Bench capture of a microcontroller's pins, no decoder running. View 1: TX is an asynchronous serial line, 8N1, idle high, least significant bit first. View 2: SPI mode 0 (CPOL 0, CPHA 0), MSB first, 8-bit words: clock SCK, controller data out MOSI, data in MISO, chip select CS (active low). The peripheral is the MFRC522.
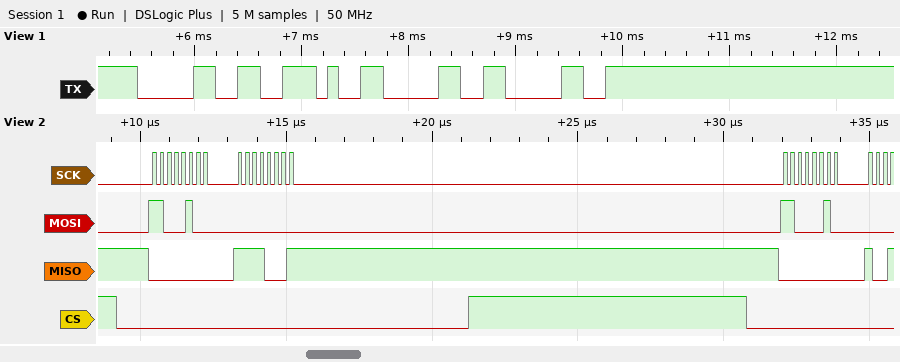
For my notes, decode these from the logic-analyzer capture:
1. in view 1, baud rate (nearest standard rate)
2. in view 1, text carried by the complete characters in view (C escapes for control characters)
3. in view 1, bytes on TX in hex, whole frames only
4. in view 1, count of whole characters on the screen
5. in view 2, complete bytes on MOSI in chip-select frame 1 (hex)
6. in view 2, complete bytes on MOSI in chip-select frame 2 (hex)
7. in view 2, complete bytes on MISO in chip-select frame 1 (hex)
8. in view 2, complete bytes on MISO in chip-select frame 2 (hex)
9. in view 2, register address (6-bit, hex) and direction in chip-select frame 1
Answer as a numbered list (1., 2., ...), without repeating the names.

1. 9600 baud
2. "0.00"
3. 30 2E 30 30
4. 4
5. C4 00
6. C2
7. 00 F1
8. 00
9. 0x22 read
